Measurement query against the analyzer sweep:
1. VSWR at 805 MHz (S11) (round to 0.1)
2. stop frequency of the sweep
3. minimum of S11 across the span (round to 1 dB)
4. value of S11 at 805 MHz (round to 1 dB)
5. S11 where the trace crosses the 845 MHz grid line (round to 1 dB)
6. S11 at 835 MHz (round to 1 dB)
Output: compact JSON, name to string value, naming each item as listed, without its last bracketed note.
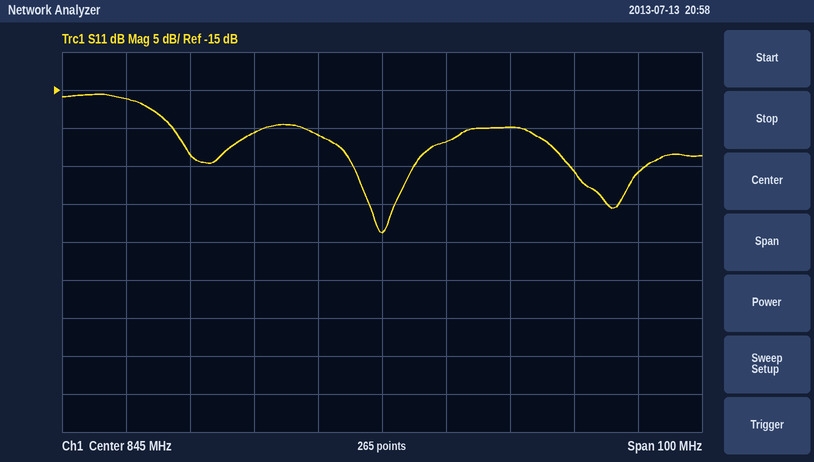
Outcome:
{"VSWR at 805 MHz (S11)": "1.4", "stop frequency of the sweep": "895 MHz", "minimum of S11 across the span": "-34 dB", "value of S11 at 805 MHz": "-16 dB", "S11 where the trace crosses the 845 MHz grid line": "-34 dB", "S11 at 835 MHz": "-21 dB"}
